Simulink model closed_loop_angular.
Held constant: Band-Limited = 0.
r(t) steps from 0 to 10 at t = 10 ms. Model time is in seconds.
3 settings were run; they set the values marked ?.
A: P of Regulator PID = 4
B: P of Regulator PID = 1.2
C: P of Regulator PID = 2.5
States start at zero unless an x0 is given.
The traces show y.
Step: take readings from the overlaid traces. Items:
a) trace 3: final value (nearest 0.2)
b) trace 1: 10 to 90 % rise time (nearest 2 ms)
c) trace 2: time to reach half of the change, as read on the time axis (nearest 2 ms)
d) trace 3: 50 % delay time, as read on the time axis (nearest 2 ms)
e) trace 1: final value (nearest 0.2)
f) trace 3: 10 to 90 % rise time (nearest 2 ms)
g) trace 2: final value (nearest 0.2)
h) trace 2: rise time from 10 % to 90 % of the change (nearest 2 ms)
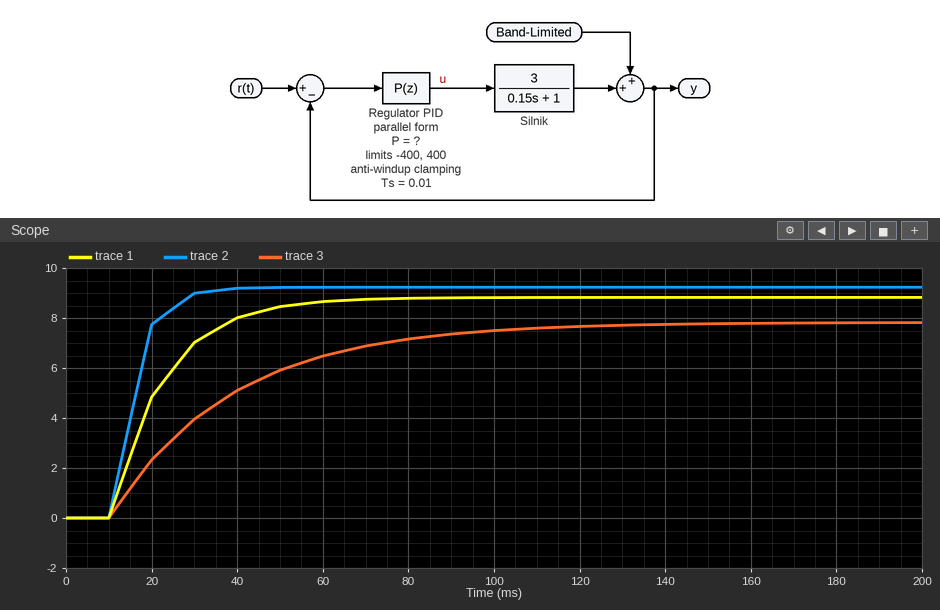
7.8
28 ms
16 ms
30 ms
8.8
62 ms
9.2
14 ms
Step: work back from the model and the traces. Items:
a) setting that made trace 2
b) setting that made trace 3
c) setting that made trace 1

A
B
C
